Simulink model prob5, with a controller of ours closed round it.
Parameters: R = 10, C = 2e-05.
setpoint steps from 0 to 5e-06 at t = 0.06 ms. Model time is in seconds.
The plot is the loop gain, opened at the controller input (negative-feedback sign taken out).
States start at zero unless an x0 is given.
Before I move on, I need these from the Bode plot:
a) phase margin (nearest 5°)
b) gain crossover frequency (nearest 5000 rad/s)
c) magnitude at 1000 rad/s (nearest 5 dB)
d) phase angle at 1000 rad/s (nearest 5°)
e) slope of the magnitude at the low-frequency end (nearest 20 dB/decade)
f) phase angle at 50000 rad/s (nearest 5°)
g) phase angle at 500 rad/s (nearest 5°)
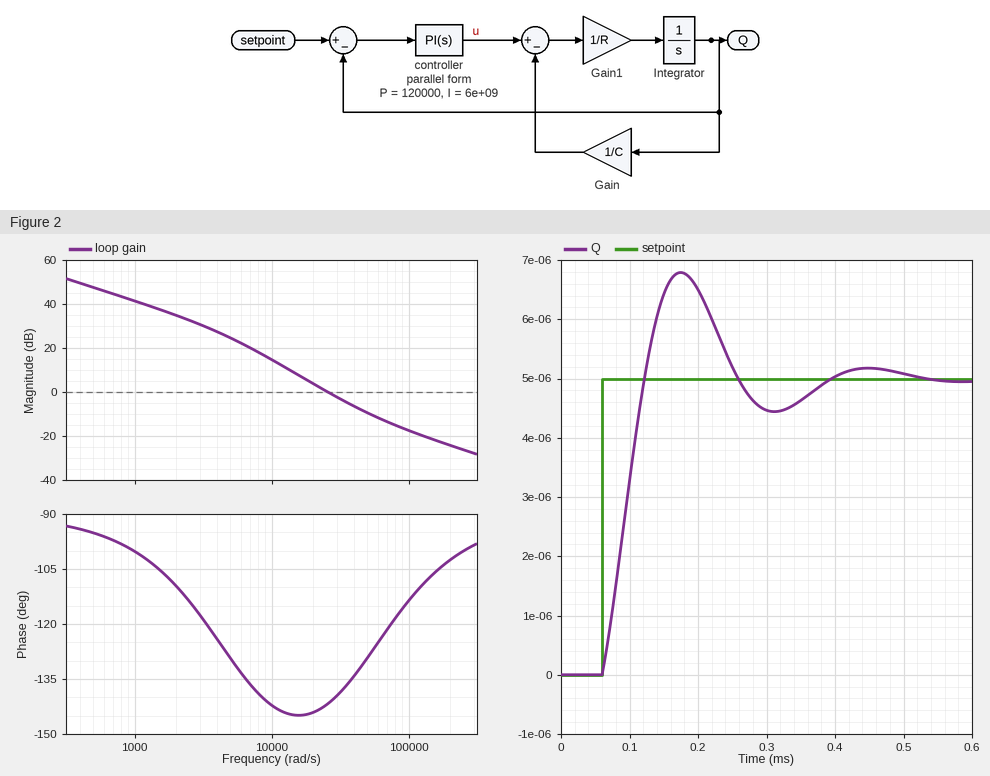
40°
25000 rad/s
40 dB
-100°
-20 dB/decade
-130°
-95°
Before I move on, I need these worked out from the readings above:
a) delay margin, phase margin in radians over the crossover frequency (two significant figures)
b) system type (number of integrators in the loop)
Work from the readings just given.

0.000028 s
1
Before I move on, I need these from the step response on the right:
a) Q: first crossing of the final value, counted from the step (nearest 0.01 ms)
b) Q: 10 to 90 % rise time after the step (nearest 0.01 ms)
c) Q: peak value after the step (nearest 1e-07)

0.06 ms
0.05 ms
0.0000068
